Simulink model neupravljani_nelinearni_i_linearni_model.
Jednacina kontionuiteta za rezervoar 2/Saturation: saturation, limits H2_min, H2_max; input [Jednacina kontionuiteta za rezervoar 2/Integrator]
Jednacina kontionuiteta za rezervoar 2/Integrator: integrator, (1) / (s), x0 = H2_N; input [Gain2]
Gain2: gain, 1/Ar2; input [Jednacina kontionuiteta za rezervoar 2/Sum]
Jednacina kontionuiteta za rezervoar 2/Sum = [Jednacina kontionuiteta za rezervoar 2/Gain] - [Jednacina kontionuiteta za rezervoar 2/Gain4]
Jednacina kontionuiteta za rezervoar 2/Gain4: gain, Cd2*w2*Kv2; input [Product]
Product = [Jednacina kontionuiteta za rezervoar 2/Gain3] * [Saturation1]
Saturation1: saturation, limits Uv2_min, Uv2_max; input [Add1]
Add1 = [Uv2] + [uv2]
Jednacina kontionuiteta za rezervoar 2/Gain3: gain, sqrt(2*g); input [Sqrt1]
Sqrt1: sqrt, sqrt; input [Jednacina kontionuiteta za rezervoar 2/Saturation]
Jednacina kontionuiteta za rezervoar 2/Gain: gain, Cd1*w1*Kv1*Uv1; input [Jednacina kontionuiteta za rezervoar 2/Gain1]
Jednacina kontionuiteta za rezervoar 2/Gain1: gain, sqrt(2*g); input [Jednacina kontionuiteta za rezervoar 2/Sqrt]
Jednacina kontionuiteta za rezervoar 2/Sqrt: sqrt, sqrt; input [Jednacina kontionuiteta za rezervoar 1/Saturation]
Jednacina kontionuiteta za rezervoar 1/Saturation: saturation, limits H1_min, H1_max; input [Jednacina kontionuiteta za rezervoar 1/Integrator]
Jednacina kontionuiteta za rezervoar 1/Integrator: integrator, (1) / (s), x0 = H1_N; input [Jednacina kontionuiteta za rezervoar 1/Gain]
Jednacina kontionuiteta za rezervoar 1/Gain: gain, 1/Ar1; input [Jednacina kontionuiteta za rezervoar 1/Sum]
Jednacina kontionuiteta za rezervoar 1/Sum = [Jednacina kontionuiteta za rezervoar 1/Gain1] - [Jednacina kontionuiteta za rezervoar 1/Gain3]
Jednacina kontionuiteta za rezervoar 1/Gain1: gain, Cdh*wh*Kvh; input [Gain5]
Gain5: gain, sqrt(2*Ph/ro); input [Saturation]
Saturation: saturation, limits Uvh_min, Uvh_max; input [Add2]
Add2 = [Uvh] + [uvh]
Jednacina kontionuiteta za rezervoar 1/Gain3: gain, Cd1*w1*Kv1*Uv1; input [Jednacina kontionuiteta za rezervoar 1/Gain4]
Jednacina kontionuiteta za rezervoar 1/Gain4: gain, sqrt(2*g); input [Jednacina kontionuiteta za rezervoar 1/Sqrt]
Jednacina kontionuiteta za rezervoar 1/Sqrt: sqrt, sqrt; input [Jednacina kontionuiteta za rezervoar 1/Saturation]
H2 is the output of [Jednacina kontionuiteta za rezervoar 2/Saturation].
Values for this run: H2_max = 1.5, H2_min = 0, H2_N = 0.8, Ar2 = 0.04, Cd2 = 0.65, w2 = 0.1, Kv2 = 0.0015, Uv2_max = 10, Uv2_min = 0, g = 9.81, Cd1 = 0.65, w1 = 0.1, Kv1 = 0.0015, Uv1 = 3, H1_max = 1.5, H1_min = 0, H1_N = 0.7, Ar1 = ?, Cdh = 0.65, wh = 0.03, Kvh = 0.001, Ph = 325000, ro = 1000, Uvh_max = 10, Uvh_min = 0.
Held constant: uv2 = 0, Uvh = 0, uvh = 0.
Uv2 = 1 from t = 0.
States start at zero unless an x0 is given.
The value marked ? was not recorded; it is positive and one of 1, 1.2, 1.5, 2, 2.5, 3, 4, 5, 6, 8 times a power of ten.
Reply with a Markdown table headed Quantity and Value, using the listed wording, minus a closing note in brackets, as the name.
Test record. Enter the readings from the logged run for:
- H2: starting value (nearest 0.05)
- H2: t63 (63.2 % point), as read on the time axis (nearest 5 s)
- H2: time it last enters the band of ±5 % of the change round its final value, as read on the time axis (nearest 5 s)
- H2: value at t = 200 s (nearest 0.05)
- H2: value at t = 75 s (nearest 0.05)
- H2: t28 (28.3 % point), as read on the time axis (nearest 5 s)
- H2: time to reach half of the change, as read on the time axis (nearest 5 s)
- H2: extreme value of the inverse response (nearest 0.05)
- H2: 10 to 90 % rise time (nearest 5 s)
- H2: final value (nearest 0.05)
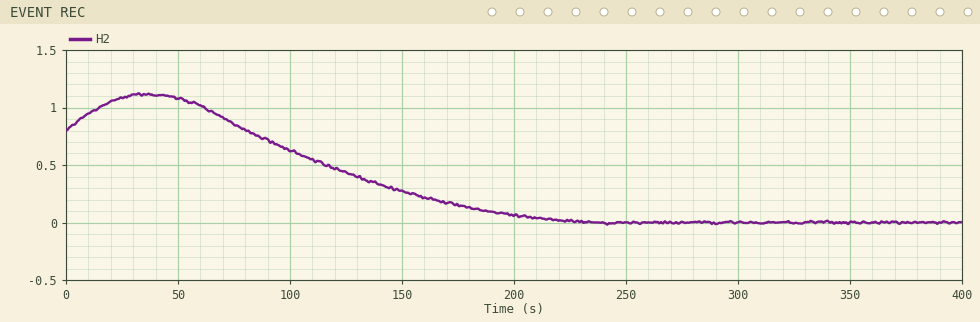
| Quantity | Value |
|---|---|
| H2: starting value | 0.80 |
| H2: t63 (63.2 % point), as read on the time axis | 145 s |
| H2: time it last enters the band of ±5 % of the change round its final value, as read on the time axis | 210 s |
| H2: value at t = 200 s | 0.05 |
| H2: value at t = 75 s | 0.85 |
| H2: t28 (28.3 % point), as read on the time axis | 105 s |
| H2: time to reach half of the change, as read on the time axis | 130 s |
| H2: extreme value of the inverse response | 1.10 |
| H2: 10 to 90 % rise time | 105 s |
| H2: final value | 0.00 |
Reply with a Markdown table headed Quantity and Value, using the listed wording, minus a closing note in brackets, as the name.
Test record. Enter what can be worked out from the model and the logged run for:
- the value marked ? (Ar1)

| Quantity | Value |
|---|---|
| the value marked ? | 0.05 |
